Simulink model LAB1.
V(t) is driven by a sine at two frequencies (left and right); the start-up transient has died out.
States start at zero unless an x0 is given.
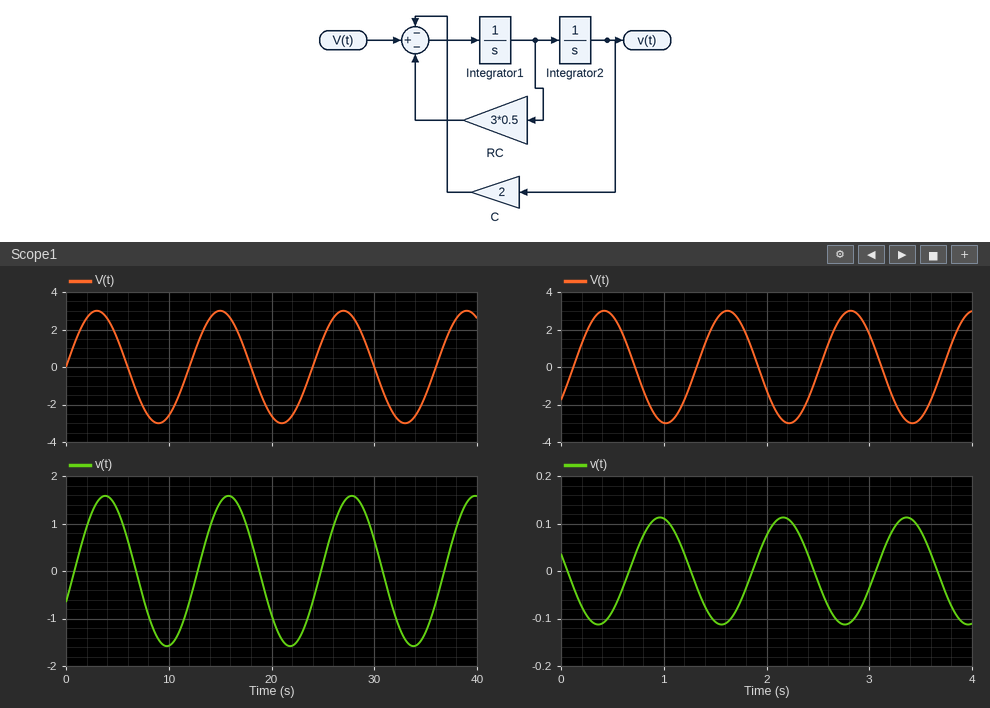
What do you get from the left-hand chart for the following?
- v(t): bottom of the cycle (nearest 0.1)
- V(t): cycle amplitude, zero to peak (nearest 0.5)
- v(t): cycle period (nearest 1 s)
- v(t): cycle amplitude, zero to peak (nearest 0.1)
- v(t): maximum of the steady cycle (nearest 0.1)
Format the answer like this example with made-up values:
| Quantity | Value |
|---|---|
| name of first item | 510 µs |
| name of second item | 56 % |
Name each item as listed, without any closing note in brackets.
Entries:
| Quantity | Value |
|---|---|
| v(t): bottom of the cycle | -1.6 |
| V(t): cycle amplitude, zero to peak | 3.0 |
| v(t): cycle period | 12 s |
| v(t): cycle amplitude, zero to peak | 1.6 |
| v(t): maximum of the steady cycle | 1.6 |
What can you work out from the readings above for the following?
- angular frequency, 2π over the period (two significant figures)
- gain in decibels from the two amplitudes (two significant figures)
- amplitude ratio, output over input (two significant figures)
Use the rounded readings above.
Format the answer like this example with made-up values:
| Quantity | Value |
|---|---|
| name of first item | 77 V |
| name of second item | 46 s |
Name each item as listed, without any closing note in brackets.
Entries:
| Quantity | Value |
|---|---|
| angular frequency, 2π over the period | 0.52 rad/s |
| gain in decibels from the two amplitudes | -5.5 dB |
| amplitude ratio, output over input | 0.53 |
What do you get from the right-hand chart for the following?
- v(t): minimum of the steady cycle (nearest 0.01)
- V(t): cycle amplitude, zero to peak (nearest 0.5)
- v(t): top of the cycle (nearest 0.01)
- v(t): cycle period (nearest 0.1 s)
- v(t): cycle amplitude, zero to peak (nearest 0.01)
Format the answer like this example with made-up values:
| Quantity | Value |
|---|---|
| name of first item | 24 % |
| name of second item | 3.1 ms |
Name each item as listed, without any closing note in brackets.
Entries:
| Quantity | Value |
|---|---|
| v(t): minimum of the steady cycle | -0.11 |
| V(t): cycle amplitude, zero to peak | 3.0 |
| v(t): top of the cycle | 0.11 |
| v(t): cycle period | 1.2 s |
| v(t): cycle amplitude, zero to peak | 0.11 |
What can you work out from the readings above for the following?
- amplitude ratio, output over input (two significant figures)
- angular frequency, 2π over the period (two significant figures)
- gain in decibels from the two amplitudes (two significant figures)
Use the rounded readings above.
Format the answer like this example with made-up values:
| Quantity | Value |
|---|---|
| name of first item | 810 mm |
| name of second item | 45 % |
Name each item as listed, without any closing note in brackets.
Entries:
| Quantity | Value |
|---|---|
| amplitude ratio, output over input | 0.037 |
| angular frequency, 2π over the period | 5.2 rad/s |
| gain in decibels from the two amplitudes | -29 dB |
